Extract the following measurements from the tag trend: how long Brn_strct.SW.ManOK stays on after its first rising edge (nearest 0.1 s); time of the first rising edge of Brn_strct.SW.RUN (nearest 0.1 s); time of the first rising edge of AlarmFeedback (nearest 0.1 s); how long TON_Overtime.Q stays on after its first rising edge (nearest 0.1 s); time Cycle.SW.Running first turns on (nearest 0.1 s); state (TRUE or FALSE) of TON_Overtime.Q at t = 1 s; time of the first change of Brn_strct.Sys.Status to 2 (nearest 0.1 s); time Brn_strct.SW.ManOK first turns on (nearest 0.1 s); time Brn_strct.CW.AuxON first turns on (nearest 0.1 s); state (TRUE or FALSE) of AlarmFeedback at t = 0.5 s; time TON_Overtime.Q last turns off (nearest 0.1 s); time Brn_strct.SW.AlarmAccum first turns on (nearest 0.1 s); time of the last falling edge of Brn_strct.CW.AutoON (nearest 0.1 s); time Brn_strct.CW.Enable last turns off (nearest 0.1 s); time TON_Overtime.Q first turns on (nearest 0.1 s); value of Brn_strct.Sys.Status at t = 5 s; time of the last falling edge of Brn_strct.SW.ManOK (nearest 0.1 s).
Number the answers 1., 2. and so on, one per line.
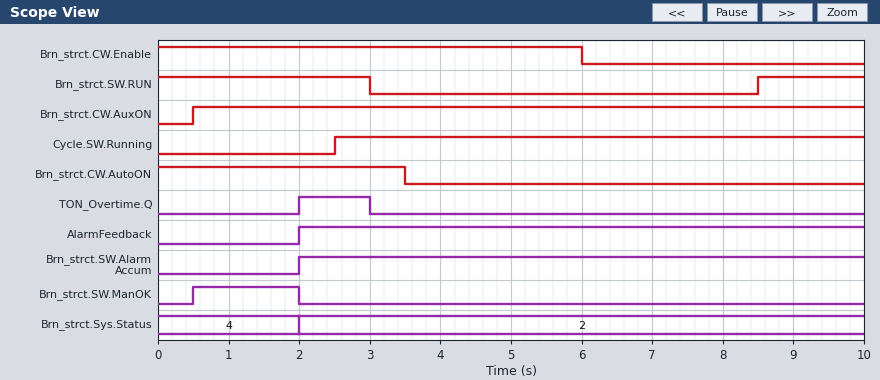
1. 1.5 s
2. 8.5 s
3. 2.0 s
4. 1.0 s
5. 2.5 s
6. FALSE
7. 2.0 s
8. 0.5 s
9. 0.5 s
10. FALSE
11. 3.0 s
12. 2.0 s
13. 3.5 s
14. 6.0 s
15. 2.0 s
16. 2
17. 2.0 s
